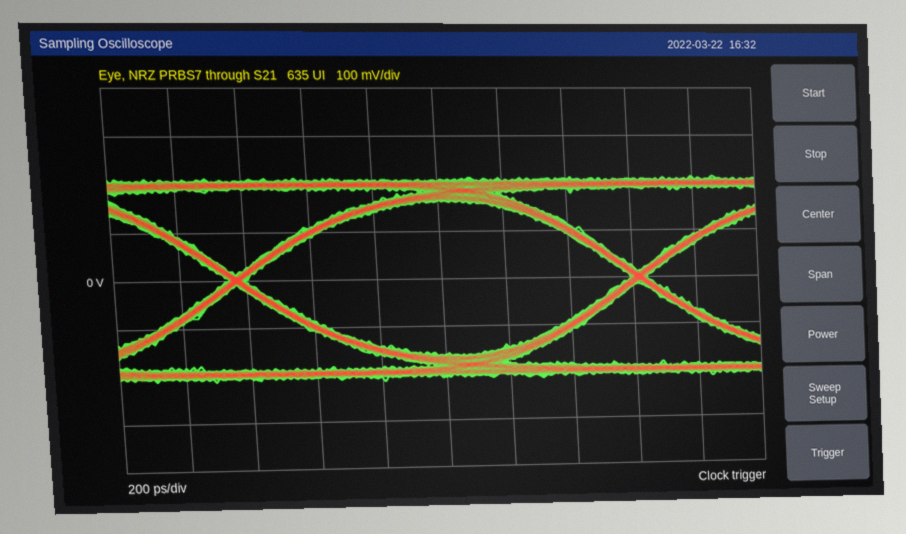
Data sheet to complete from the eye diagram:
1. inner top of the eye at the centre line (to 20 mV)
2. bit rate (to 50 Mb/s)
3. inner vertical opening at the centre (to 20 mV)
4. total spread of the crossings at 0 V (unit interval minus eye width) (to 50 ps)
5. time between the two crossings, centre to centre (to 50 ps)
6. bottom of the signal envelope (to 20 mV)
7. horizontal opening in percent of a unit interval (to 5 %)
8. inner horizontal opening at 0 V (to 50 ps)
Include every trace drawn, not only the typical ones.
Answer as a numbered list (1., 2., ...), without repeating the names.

1. 160 mV
2. 800 Mb/s
3. 320 mV
4. 50 ps
5. 1.25 ns
6. -220 mV
7. 95 %
8. 1.20 ns
